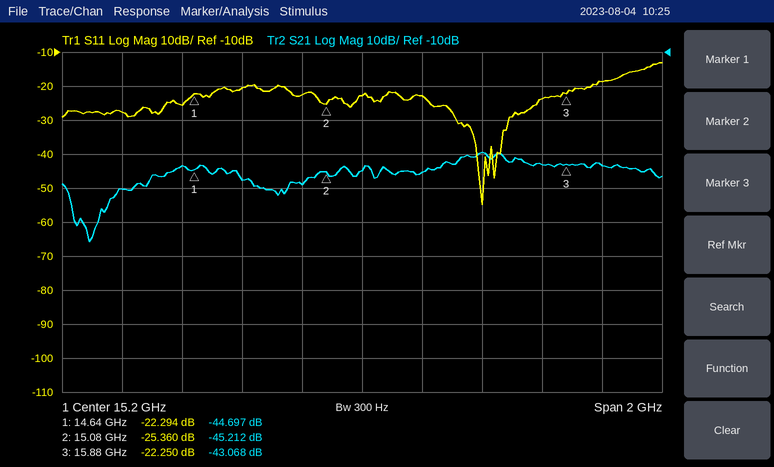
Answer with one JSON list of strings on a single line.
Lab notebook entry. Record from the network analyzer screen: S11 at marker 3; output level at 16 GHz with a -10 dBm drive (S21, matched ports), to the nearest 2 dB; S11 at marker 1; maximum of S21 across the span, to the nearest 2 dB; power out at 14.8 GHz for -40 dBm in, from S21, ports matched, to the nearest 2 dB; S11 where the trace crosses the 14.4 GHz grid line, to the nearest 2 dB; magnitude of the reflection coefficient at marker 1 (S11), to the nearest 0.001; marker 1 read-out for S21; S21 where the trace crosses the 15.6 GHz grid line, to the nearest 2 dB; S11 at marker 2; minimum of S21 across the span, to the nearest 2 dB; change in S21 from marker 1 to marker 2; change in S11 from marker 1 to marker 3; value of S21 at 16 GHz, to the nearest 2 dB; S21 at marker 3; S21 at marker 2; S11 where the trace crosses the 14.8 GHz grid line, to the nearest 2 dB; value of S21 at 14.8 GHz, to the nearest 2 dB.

["-22.250 dB", "-54 dBm", "-22.294 dB", "-40 dB", "-88 dBm", "-28 dB", "0.077", "-44.697 dB", "-40 dB", "-25.360 dB", "-66 dB", "-0.515 dB", "0.044 dB", "-44 dB", "-43.068 dB", "-45.212 dB", "-20 dB", "-48 dB"]
